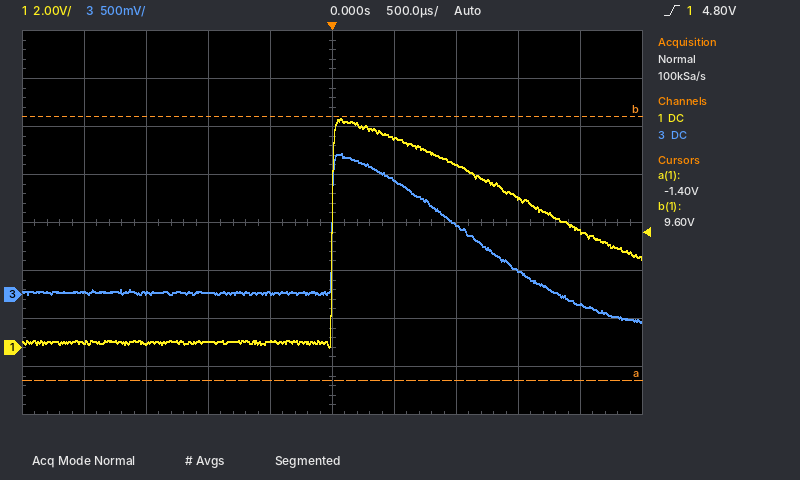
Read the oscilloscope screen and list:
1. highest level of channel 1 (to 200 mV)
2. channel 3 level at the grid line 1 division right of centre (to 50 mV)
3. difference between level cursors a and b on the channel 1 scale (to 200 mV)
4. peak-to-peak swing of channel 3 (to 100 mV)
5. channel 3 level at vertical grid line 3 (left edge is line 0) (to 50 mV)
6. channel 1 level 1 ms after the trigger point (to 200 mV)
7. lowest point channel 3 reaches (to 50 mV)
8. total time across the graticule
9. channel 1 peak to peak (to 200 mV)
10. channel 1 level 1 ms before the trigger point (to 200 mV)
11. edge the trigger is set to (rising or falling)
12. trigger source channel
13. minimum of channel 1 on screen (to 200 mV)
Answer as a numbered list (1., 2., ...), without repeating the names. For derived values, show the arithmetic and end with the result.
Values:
1. 9.6 V
2. 1.20 V
3. 11.0 V
4. 1.80 V
5. 0 mV
6. 7.6 V
7. -300 mV
8. 5 ms
9. 9.6 V − (0.0 V) = 9.6 V
10. 200 mV
11. rising
12. channel 1
13. 0.0 V
